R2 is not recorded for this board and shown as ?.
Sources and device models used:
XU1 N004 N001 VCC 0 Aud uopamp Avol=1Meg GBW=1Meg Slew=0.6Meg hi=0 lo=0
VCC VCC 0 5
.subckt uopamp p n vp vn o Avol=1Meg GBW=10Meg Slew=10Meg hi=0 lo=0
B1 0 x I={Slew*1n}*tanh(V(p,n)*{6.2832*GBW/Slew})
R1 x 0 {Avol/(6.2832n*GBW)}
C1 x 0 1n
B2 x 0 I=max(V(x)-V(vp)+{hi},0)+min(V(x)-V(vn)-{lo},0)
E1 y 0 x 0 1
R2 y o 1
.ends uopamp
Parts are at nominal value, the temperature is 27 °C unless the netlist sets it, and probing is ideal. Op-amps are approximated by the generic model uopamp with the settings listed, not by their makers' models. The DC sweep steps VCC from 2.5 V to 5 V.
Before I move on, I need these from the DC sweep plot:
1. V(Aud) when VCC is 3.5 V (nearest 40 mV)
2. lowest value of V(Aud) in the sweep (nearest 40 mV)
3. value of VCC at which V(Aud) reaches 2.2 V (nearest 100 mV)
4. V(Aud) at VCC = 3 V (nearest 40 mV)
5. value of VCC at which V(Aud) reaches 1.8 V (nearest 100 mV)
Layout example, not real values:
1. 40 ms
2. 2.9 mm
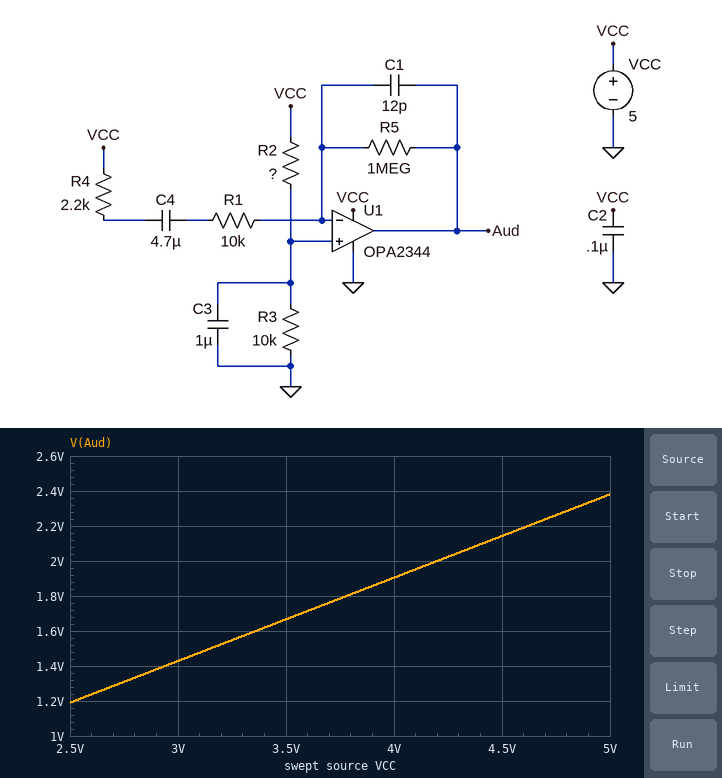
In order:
1. 1.68 V
2. 1.20 V
3. 4.6 V
4. 1.44 V
5. 3.8 V
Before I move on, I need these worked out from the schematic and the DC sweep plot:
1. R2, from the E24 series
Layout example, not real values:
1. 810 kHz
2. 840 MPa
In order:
1. 11 kΩ
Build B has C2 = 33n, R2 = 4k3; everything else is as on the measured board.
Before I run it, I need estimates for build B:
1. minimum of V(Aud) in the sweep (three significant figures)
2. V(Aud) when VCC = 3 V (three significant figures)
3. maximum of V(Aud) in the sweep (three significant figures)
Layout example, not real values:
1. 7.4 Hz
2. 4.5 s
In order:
1. 1.75 V
2. 2.10 V
3. 3.50 V
